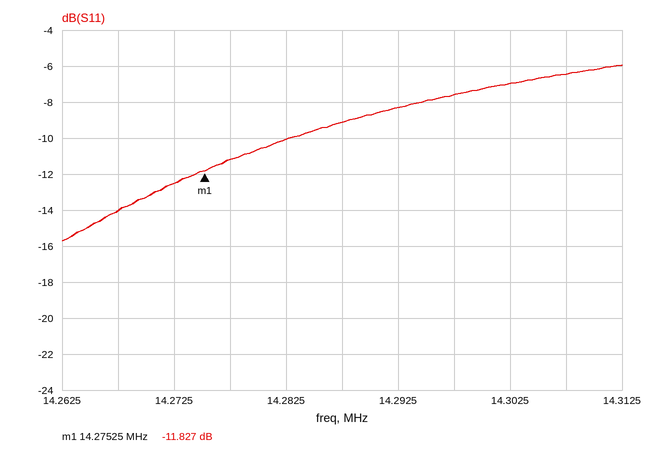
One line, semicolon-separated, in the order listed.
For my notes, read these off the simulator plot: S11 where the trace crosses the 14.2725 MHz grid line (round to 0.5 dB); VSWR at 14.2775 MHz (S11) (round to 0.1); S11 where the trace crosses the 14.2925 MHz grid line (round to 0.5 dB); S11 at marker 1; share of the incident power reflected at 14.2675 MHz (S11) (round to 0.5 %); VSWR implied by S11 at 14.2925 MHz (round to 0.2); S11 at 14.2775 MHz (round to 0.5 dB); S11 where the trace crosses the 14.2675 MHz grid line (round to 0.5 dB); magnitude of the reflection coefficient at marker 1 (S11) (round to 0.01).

-12.5 dB; 1.8; -8.5 dB; -11.827 dB; 4.0 %; 2.2; -11.0 dB; -14.0 dB; 0.26
